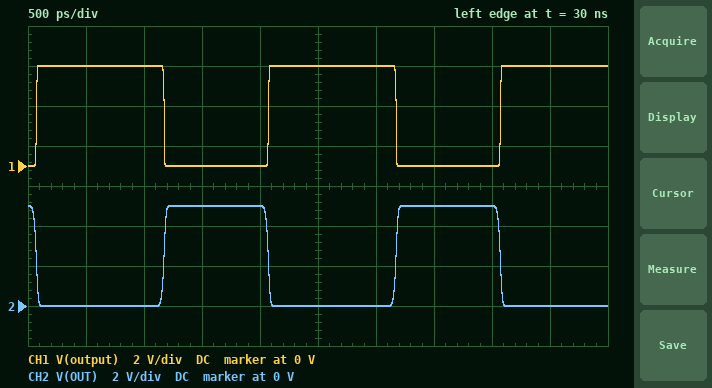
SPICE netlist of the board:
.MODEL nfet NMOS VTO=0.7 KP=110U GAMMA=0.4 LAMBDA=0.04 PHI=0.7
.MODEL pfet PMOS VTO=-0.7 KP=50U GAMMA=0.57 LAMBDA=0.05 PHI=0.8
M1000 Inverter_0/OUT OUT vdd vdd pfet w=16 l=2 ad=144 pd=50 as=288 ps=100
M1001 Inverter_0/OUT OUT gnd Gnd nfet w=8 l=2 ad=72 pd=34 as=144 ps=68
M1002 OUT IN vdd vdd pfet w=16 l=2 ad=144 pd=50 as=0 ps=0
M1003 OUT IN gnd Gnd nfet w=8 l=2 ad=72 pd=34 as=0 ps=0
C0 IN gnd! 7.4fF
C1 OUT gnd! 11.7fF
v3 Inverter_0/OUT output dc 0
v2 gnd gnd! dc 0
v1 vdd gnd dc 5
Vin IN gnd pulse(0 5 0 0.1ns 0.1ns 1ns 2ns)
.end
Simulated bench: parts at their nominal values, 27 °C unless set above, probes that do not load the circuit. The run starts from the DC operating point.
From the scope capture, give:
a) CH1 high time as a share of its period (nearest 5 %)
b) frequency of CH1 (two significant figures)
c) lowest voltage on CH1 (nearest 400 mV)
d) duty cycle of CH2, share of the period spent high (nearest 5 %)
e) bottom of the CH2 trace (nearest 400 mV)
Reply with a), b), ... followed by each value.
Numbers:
a) 55 %
b) 500 MHz
c) 0 V
d) 45 %
e) 0 V
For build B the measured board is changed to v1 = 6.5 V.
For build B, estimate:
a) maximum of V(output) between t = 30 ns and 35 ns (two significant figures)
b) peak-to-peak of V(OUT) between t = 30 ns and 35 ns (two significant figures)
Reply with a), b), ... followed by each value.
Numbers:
a) 6.5 V
b) 6.4 V
